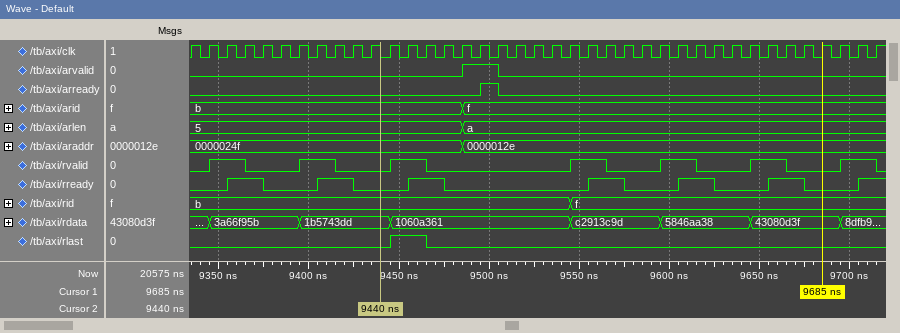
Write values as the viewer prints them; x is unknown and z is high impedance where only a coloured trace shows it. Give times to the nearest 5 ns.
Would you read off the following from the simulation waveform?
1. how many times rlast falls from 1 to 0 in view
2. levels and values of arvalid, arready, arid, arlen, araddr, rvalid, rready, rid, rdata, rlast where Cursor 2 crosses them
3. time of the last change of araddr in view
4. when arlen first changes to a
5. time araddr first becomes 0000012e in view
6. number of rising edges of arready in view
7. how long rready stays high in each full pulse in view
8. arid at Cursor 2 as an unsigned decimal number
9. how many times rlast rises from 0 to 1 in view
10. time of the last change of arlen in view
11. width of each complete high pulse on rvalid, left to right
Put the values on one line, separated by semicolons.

1; arvalid=0, arready=0, arid=b, arlen=5, araddr=0000024f, rvalid=0, rready=0, rid=b, rdata=1b5743dd, rlast=0; 9485 ns; 9485 ns; 9485 ns; 1; 20 ns, 20 ns, 20 ns, 20 ns, 20 ns, 20 ns; 11; 1; 9485 ns; 20 ns, 20 ns, 20 ns, 20 ns, 20 ns, 20 ns, 20 ns
